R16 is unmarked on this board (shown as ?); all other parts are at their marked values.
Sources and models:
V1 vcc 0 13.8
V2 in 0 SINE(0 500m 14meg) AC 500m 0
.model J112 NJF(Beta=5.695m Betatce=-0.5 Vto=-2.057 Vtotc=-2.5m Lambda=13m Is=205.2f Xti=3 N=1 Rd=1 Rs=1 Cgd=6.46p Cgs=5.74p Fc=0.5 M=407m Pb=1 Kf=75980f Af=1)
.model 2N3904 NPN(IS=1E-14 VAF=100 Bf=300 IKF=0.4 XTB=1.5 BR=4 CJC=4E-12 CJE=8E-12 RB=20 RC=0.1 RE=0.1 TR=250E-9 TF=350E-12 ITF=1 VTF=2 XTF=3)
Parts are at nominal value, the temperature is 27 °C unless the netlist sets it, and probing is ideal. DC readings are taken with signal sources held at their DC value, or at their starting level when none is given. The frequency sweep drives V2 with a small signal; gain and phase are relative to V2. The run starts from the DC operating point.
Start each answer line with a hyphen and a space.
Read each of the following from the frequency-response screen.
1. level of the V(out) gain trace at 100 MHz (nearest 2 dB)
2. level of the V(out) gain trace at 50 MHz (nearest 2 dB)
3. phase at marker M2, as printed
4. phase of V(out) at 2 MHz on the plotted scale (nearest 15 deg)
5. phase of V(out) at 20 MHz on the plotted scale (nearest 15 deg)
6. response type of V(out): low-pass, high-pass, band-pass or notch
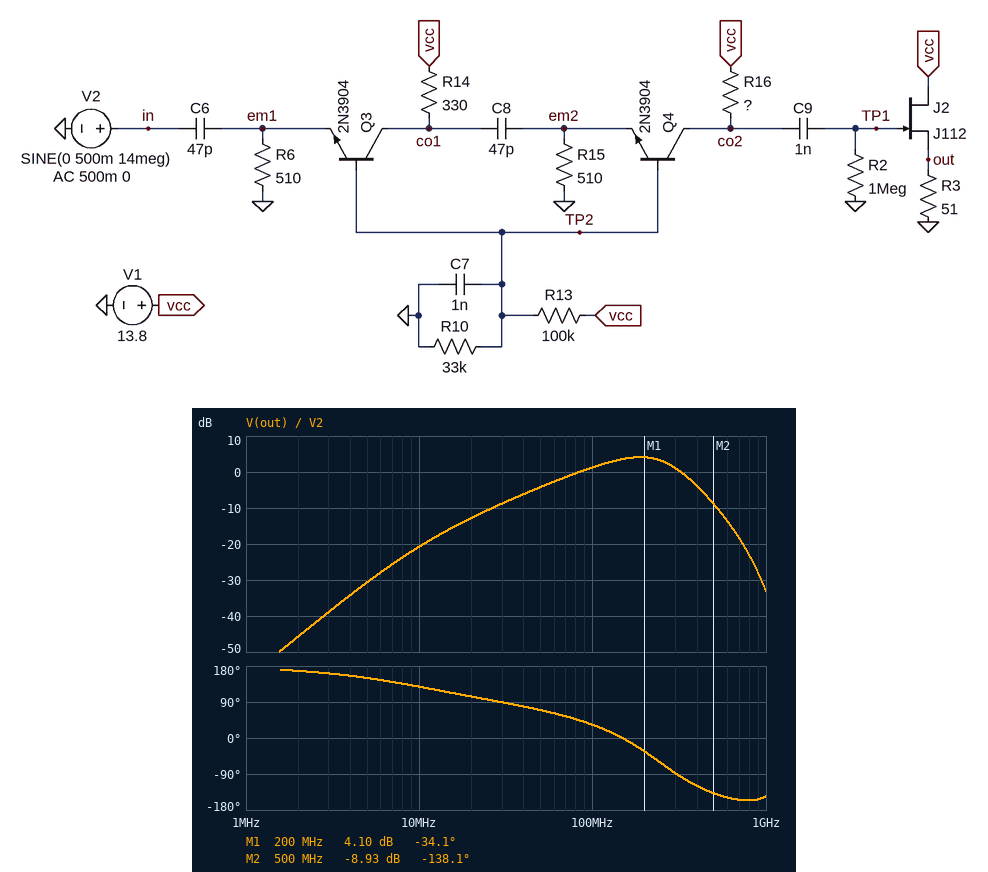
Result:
- 2 dB
- -4 dB
- -138.1 deg
- 165 deg
- 105 deg
- band-pass
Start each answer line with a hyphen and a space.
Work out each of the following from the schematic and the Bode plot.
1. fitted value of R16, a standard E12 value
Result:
- 100 Ω
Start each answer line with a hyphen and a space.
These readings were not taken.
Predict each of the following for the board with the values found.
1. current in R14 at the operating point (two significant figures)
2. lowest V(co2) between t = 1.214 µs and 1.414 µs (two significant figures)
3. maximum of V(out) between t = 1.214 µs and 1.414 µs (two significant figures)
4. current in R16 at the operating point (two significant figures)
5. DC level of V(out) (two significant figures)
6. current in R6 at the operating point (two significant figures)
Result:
- 4.1 mA
- 13 V
- 730 mV
- 4.1 mA
- 660 mV
- 4.1 mA
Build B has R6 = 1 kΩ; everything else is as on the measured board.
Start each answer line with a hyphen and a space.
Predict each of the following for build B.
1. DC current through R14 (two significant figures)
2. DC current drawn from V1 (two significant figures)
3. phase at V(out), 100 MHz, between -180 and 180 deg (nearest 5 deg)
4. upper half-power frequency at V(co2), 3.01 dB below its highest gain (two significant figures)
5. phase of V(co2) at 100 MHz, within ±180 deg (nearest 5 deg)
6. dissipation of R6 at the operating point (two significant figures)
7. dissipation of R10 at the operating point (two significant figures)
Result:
- 2.2 mA
- 20 mA
- 25 deg
- 270 MHz
- 20 deg
- 5.1 mW
- 260 µW
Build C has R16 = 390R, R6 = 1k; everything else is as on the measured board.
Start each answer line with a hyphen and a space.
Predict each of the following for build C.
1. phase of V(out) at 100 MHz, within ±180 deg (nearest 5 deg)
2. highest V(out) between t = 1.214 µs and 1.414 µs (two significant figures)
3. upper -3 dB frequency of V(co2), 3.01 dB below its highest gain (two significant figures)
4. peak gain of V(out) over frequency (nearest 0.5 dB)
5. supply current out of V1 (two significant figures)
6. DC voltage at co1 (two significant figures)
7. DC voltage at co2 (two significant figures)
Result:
- -10 deg
- 930 mV
- 210 MHz
- 8.0 dB
- 20 mA
- 13 V
- 12 V
